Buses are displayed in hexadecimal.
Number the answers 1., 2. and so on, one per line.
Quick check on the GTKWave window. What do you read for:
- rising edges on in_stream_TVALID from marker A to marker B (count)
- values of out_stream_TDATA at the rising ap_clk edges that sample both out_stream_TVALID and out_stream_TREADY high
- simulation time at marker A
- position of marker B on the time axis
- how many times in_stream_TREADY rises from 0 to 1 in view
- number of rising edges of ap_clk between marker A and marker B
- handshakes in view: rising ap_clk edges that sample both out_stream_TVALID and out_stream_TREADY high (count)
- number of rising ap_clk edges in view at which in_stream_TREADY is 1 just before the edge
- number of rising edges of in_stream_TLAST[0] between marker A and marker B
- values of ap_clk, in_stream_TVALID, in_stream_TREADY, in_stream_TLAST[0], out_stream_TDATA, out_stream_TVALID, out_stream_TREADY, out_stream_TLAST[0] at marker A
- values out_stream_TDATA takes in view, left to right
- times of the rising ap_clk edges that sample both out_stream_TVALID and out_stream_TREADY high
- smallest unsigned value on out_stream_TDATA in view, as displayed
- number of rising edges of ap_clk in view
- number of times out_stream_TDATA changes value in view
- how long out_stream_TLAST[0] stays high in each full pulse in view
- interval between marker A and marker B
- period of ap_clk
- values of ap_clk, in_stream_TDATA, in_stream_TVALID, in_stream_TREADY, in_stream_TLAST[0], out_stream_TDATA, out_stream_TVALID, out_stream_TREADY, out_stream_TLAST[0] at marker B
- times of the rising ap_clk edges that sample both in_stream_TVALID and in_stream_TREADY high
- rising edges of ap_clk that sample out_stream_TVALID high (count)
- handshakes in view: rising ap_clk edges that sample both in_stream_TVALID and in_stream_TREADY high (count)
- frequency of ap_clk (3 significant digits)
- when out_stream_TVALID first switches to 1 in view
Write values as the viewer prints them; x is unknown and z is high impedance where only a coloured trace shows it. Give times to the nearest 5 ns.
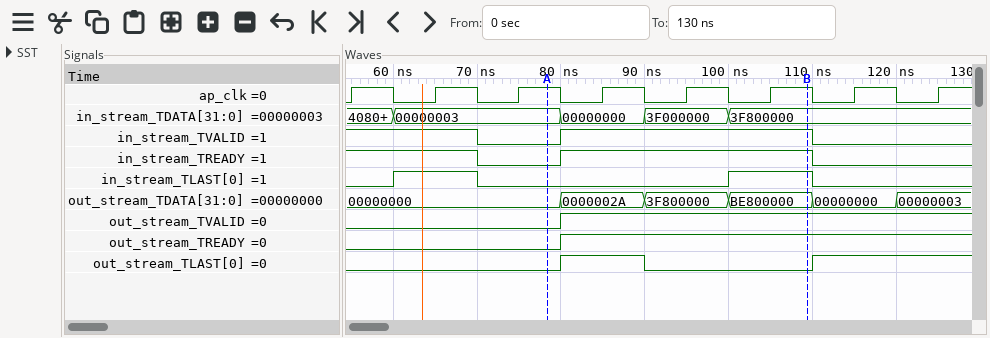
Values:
1. 1
2. 0000002A, 3F800000, BE800000, 00000000, 00000003
3. 80 ns
4. 110 ns
5. 1
6. 3
7. 5
8. 5
9. 1
10. ap_clk=1, in_stream_TVALID=0, in_stream_TREADY=0, in_stream_TLAST[0]=0, out_stream_TDATA=00000000, out_stream_TVALID=0, out_stream_TREADY=0, out_stream_TLAST[0]=0
11. 00000000, 0000002A, 3F800000, BE800000, 00000000, 00000003
12. 85 ns, 95 ns, 105 ns, 115 ns, 125 ns
13. 00000000
14. 8
15. 5
16. 10 ns
17. 30 ns
18. 10 ns
19. ap_clk=1, in_stream_TDATA=3F800000, in_stream_TVALID=1, in_stream_TREADY=1, in_stream_TLAST[0]=1, out_stream_TDATA=BE800000, out_stream_TVALID=1, out_stream_TREADY=1, out_stream_TLAST[0]=0
20. 55 ns, 65 ns, 85 ns, 95 ns, 105 ns
21. 5
22. 5
23. 100 MHz
24. 80 ns
